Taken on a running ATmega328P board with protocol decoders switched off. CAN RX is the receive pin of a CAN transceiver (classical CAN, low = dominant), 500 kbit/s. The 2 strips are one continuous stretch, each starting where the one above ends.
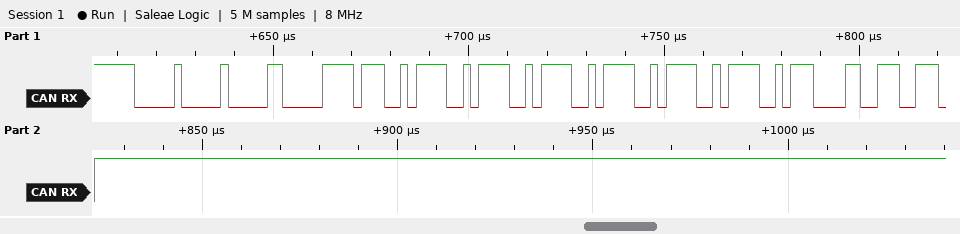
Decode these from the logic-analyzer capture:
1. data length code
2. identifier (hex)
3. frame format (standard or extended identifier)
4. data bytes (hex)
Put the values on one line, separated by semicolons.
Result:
8; 0x000; standard; 3B 97 97 97 97 97 97 97
